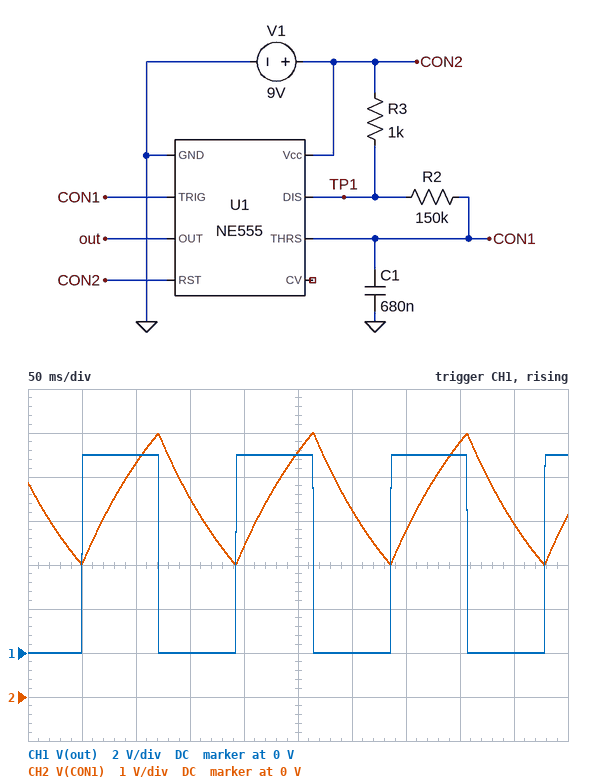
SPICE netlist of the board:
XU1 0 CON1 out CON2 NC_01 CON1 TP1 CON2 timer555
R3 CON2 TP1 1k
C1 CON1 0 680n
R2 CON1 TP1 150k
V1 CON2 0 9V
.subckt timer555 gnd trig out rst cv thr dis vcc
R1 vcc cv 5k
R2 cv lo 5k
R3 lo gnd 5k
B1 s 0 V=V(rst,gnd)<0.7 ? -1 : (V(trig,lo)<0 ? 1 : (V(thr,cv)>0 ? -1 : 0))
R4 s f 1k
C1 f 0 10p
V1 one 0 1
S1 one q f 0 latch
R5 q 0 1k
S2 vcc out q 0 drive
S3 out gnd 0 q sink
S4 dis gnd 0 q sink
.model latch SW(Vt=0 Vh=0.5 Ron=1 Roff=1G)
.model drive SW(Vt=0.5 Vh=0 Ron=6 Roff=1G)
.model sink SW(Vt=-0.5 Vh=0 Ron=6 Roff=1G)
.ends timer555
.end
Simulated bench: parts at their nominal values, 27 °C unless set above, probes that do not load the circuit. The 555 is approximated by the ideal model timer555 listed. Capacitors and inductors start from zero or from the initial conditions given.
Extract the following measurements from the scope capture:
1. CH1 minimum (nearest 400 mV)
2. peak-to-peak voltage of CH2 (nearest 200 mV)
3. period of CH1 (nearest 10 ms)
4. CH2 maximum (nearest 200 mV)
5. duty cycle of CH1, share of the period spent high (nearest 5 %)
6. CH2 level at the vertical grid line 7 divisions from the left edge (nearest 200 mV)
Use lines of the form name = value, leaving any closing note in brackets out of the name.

CH1 minimum = 0 V
peak-to-peak voltage of CH2 = 3.0 V
period of CH1 = 140 ms
CH2 maximum = 6.0 V
duty cycle of CH1, share of the period spent high = 50 %
CH2 level at the vertical grid line 7 divisions from the left edge = 3.8 V
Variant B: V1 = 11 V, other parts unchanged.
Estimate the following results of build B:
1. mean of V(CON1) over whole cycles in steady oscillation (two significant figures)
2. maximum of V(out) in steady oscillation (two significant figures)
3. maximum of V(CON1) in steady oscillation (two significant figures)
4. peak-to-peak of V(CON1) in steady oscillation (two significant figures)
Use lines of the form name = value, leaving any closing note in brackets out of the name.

mean of V(CON1) over whole cycles in steady oscillation = 5.5 V
maximum of V(out) in steady oscillation = 11 V
maximum of V(CON1) in steady oscillation = 7.3 V
peak-to-peak of V(CON1) in steady oscillation = 3.7 V
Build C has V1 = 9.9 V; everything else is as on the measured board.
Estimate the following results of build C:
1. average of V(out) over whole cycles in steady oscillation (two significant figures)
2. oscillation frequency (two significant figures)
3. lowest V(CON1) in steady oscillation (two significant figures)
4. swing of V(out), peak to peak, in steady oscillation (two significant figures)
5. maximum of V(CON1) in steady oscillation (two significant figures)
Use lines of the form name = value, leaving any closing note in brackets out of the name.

average of V(out) over whole cycles in steady oscillation = 4.9 V
oscillation frequency = 7.0 Hz
lowest V(CON1) in steady oscillation = 3.3 V
swing of V(out), peak to peak, in steady oscillation = 9.9 V
maximum of V(CON1) in steady oscillation = 6.6 V
